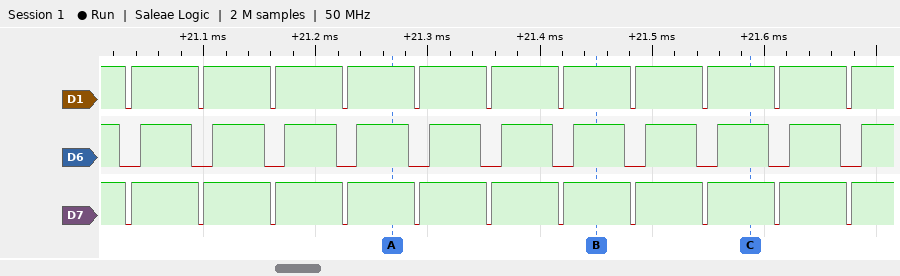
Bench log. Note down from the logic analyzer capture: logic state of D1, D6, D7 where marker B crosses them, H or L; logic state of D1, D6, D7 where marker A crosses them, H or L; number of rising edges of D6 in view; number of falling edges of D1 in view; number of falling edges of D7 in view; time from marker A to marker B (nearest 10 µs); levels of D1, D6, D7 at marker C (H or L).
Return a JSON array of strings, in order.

["D1=H, D6=H, D7=H", "D1=H, D6=H, D7=H", "11", "11", "11", "180 µs", "D1=H, D6=H, D7=H"]
